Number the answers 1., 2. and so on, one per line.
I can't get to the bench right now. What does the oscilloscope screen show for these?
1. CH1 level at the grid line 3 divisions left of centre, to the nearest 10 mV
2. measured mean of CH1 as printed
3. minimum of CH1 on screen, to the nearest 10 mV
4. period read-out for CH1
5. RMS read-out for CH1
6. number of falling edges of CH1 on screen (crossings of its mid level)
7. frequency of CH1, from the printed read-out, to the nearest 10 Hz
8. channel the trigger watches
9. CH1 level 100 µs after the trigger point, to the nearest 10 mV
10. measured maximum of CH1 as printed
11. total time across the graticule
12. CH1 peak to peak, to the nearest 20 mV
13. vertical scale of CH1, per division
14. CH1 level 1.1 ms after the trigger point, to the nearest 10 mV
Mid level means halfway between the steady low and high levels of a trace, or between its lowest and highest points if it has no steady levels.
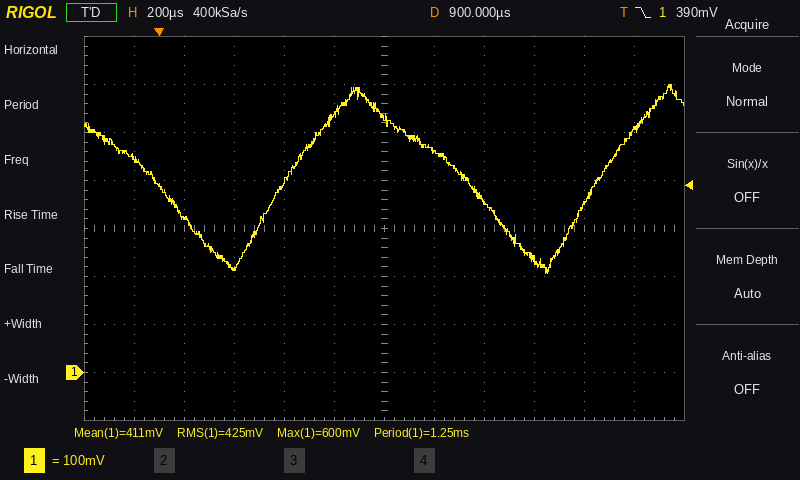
1. 220 mV
2. 411 mV
3. 210 mV
4. 1.25 ms
5. 425 mV
6. 2
7. 800 Hz
8. CH1
9. 320 mV
10. 600 mV
11. 2.4 ms
12. 400 mV
13. 100 mV
14. 460 mV
